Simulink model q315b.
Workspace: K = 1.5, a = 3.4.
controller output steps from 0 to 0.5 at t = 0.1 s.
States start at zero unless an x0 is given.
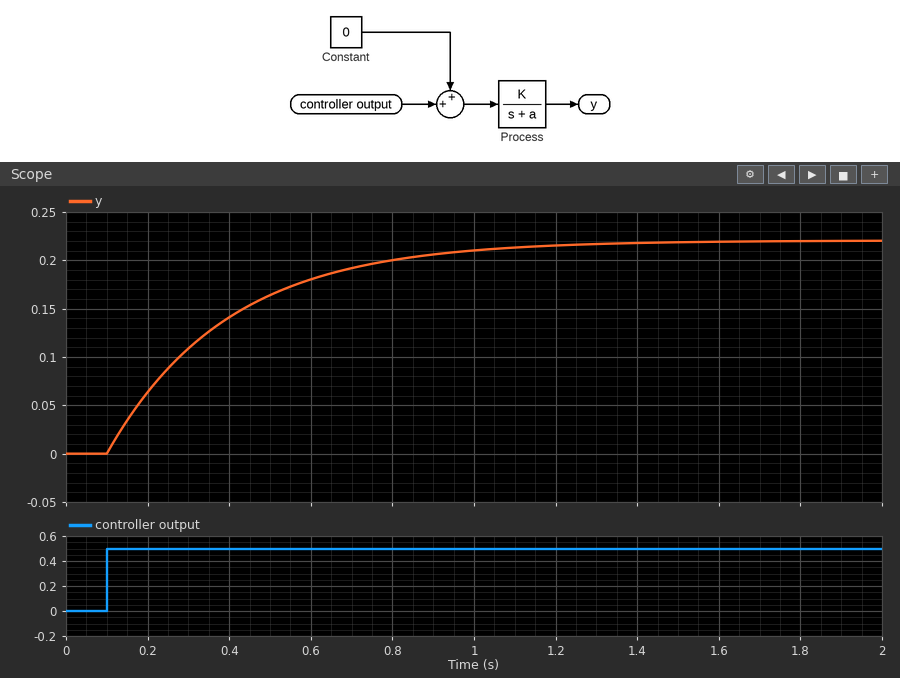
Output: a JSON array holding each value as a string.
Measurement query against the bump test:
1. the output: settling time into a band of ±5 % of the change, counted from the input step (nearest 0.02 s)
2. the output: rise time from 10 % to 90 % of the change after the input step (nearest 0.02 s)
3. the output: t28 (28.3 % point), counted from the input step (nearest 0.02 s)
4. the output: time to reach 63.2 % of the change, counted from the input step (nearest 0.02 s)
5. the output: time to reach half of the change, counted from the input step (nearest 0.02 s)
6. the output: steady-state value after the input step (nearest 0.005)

["0.88 s", "0.64 s", "0.10 s", "0.30 s", "0.20 s", "0.220"]
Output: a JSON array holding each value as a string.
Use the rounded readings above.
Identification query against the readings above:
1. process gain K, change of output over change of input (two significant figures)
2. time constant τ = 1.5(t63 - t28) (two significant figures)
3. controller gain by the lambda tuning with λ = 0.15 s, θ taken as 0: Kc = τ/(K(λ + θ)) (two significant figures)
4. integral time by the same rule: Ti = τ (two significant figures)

["0.44", "0.30 s", "4.5", "0.30 s"]
